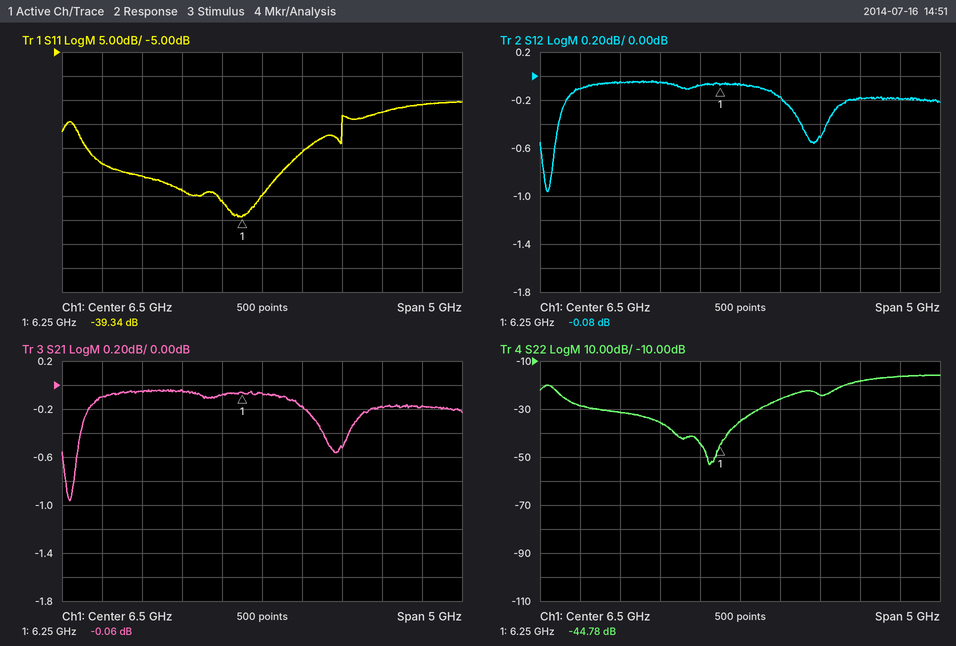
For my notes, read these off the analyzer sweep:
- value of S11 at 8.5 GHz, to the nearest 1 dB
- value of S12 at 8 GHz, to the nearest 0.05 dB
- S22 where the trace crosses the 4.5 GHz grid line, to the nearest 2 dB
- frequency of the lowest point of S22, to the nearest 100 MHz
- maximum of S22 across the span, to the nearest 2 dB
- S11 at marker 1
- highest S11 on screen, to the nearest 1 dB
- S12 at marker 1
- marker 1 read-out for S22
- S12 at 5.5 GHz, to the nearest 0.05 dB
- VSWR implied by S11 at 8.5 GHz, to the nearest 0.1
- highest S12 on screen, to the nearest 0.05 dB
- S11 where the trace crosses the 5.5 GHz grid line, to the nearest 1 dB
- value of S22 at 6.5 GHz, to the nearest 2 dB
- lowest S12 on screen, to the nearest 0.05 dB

-16 dB
-0.20 dB
-28 dB
6.1 GHz
-16 dB
-39.34 dB
-15 dB
-0.08 dB
-44.78 dB
-0.05 dB
1.4
-0.05 dB
-34 dB
-36 dB
-0.95 dB
